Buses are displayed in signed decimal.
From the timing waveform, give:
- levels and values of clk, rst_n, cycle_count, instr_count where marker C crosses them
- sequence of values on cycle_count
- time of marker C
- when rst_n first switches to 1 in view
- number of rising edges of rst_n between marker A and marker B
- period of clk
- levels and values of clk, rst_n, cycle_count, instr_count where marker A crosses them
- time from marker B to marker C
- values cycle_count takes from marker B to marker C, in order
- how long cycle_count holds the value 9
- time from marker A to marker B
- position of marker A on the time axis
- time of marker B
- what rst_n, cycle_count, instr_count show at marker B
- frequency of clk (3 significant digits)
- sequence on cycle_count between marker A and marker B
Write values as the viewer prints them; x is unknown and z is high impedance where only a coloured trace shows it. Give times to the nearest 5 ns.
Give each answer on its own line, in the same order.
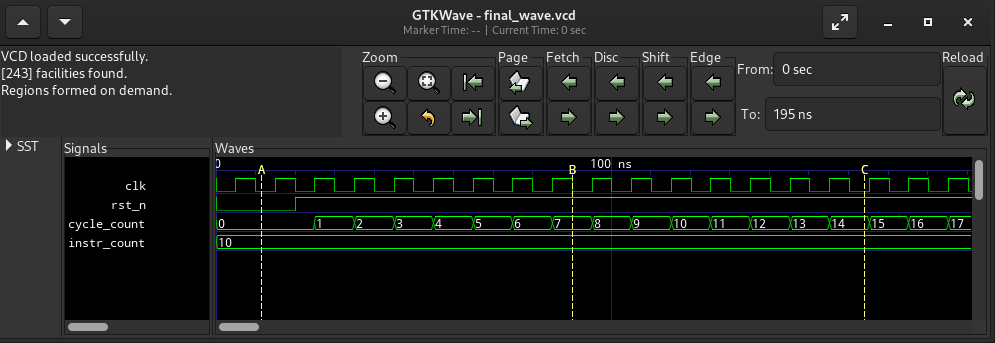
clk=0, rst_n=1, cycle_count=14, instr_count=10
0, 1, 2, 3, 4, 5, 6, 7, 8, 9, 10, 11, 12, 13, 14, 15, 16, 17
165 ns
20 ns
1
10 ns
clk=0, rst_n=0, cycle_count=0, instr_count=10
75 ns
7, 8, 9, 10, 11, 12, 13, 14
10 ns
80 ns
10 ns
90 ns
rst_n=1, cycle_count=7, instr_count=10
100 MHz
0, 1, 2, 3, 4, 5, 6, 7
